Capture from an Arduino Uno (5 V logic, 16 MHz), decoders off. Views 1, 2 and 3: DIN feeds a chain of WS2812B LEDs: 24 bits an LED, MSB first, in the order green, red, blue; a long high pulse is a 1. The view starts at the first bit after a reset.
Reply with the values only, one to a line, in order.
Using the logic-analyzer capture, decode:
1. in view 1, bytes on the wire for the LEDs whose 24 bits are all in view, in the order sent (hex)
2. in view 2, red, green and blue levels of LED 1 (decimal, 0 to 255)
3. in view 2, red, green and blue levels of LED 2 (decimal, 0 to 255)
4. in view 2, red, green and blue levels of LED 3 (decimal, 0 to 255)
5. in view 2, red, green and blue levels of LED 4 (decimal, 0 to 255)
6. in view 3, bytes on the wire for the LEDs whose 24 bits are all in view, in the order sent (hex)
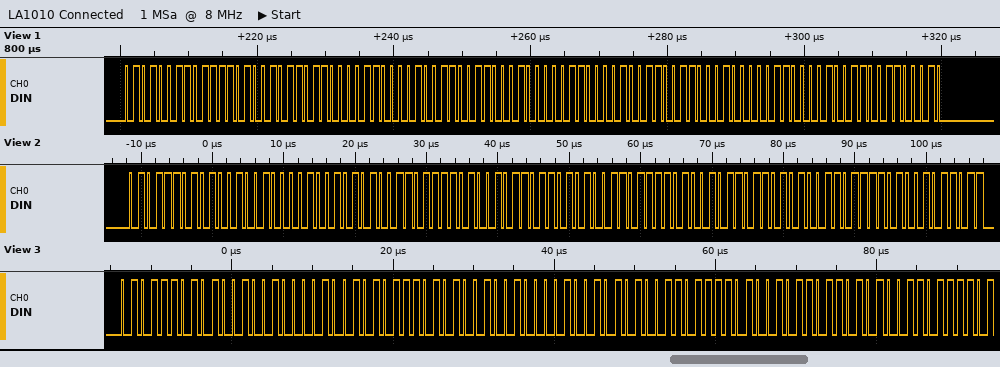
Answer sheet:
53 7A 5B 0C 26 62 0C 26 62 0C 26 62
73, 93, 9
122, 83, 91
122, 83, 91
122, 83, 91
5D 49 09 5D 49 09 53 7A 5B
